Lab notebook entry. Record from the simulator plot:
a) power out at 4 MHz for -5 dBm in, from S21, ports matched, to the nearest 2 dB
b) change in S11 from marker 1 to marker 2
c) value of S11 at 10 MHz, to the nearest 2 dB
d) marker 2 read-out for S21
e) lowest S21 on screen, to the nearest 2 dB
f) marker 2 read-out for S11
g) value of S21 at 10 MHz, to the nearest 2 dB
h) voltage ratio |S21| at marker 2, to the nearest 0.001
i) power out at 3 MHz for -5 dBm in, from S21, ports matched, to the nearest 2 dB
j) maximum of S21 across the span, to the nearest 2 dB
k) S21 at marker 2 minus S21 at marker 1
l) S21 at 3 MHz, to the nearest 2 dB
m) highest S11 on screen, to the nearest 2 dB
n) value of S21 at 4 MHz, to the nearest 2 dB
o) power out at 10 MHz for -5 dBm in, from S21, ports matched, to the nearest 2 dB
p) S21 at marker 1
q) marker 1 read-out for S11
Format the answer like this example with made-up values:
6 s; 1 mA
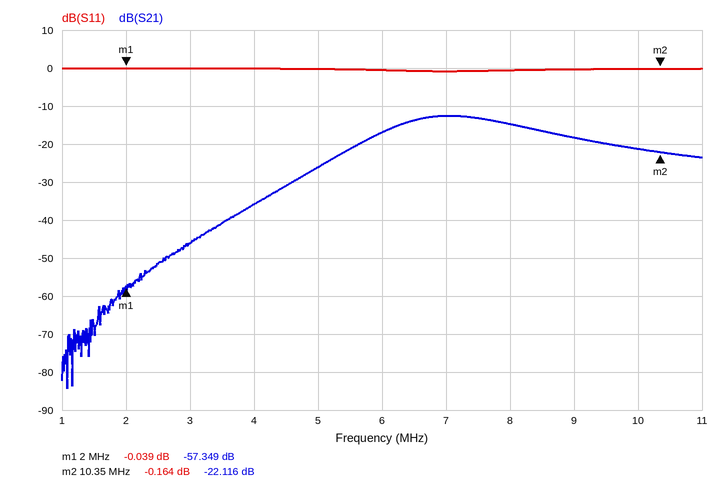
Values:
-40 dBm; -0.125 dB; 0 dB; -22.116 dB; -84 dB; -0.164 dB; -22 dB; 0.078; -52 dBm; -12 dB; 35.233 dB; -46 dB; 0 dB; -36 dB; -26 dBm; -57.349 dB; -0.039 dB
